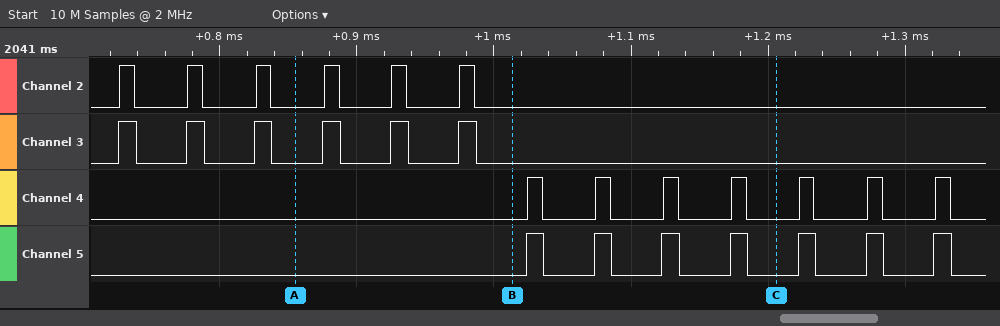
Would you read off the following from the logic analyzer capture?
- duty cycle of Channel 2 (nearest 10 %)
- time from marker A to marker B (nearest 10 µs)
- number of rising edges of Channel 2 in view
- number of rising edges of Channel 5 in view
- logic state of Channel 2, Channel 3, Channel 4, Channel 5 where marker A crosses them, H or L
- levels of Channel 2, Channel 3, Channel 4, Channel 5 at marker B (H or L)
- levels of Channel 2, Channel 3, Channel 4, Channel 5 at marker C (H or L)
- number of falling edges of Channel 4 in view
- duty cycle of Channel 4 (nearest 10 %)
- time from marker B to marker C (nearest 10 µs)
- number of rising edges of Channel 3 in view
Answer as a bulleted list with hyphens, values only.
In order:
- 20 %
- 160 µs
- 6
- 7
- Channel 2=L, Channel 3=L, Channel 4=L, Channel 5=L
- Channel 2=L, Channel 3=L, Channel 4=L, Channel 5=L
- Channel 2=L, Channel 3=L, Channel 4=L, Channel 5=L
- 7
- 20 %
- 190 µs
- 6
